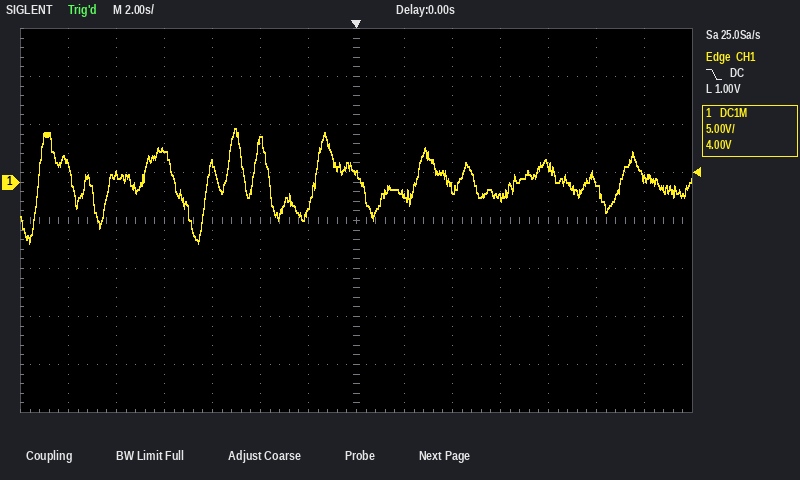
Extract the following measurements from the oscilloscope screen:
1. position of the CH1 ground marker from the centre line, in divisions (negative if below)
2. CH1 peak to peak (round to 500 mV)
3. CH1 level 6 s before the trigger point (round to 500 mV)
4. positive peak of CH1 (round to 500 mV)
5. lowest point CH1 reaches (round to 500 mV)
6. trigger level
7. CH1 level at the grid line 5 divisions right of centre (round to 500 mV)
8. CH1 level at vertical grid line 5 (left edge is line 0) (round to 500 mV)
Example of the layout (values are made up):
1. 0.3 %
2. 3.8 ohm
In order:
1. +0.8 div
2. 12.0 V
3. 2.0 V
4. 5.5 V
5. -6.5 V
6. 1.00 V
7. 0.0 V
8. 4.5 V
